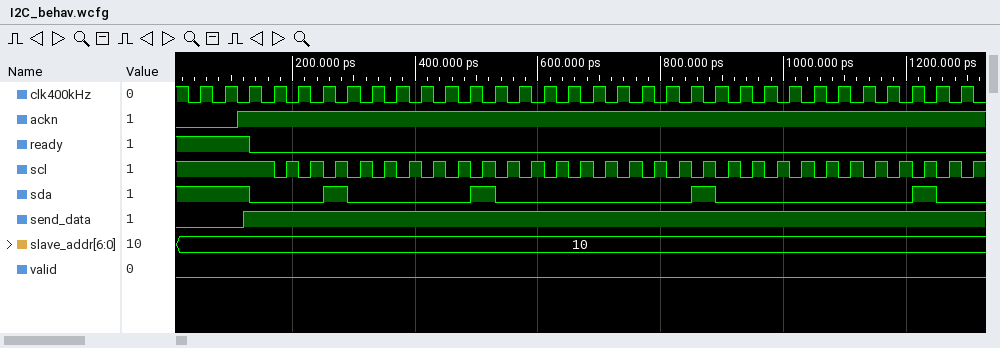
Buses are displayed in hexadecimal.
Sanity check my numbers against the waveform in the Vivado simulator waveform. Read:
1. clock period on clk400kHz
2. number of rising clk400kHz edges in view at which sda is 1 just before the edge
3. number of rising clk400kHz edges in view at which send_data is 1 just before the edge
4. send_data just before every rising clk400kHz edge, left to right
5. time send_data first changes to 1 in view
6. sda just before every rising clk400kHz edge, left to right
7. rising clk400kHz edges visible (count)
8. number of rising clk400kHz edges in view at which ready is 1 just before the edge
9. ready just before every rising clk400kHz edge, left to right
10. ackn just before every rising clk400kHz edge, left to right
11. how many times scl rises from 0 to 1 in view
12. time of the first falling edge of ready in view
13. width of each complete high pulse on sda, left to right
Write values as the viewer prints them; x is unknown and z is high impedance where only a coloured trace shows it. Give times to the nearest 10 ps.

40 ps
7
30
0 0 1 1 1 1 1 1 1 1 1 1 1 1 1 1 1 1 1 1 1 1 1 1 1 1 1 1 1 1 1 1
120 ps
1 1 1 0 0 0 1 0 0 0 0 0 1 0 0 0 0 0 0 0 0 1 0 0 0 0 0 0 0 0 1 0
32
3
1 1 1 0 0 0 0 0 0 0 0 0 0 0 0 0 0 0 0 0 0 0 0 0 0 0 0 0 0 0 0 0
0 0 1 1 1 1 1 1 1 1 1 1 1 1 1 1 1 1 1 1 1 1 1 1 1 1 1 1 1 1 1 1
29
130 ps
40 ps, 40 ps, 40 ps, 40 ps
